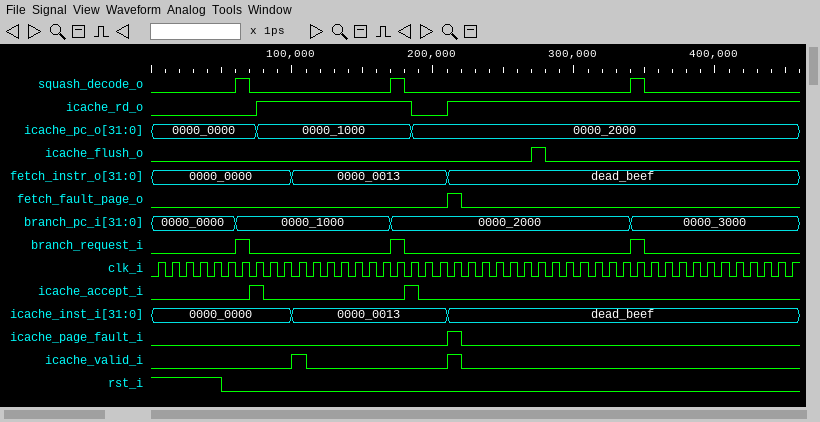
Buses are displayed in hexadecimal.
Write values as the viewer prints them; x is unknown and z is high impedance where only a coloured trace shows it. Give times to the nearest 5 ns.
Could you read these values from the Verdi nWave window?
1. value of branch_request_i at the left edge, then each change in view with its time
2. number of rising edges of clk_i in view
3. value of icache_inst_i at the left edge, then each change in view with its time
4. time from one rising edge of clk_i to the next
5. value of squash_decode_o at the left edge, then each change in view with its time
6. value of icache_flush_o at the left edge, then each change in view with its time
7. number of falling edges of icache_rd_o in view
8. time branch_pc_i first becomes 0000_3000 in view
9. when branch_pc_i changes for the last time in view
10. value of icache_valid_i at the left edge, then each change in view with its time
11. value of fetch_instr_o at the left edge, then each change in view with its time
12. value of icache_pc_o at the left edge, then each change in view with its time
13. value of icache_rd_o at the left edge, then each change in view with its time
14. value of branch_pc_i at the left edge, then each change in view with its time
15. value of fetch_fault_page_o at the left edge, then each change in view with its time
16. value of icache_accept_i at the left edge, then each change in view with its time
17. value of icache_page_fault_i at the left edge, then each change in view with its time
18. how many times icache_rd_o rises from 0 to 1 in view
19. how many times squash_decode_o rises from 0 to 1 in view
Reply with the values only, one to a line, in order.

0, 1 at 60 ns, 0 at 70 ns, 1 at 170 ns, 0 at 180 ns, 1 at 340 ns, 0 at 350 ns
46
0000_0000, 0000_0013 at 100 ns, dead_beef at 210 ns
10 ns
0, 1 at 60 ns, 0 at 70 ns, 1 at 170 ns, 0 at 180 ns, 1 at 340 ns, 0 at 350 ns
0, 1 at 270 ns, 0 at 280 ns
1
340 ns
340 ns
0, 1 at 100 ns, 0 at 110 ns, 1 at 210 ns, 0 at 220 ns
0000_0000, 0000_0013 at 100 ns, dead_beef at 210 ns
0000_0000, 0000_1000 at 75 ns, 0000_2000 at 185 ns
0, 1 at 75 ns, 0 at 185 ns, 1 at 210 ns
0000_0000, 0000_1000 at 60 ns, 0000_2000 at 170 ns, 0000_3000 at 340 ns
0, 1 at 210 ns, 0 at 220 ns
0, 1 at 70 ns, 0 at 80 ns, 1 at 180 ns, 0 at 190 ns
0, 1 at 210 ns, 0 at 220 ns
2
3
